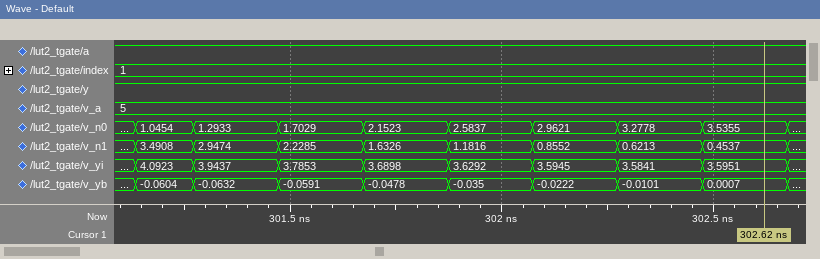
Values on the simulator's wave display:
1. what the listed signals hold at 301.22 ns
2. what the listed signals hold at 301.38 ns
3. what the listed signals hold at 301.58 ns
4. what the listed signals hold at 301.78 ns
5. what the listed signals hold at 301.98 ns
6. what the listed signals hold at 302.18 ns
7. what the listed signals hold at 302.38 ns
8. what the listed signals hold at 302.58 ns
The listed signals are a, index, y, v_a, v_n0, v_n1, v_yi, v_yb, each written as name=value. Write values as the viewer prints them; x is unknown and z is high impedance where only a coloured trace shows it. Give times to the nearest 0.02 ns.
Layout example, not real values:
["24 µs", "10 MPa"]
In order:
["a=1, index=1, y=1, v_a=5, v_n0=1.0454, v_n1=3.4908, v_yi=4.0923, v_yb=-0.0604", "a=1, index=1, y=1, v_a=5, v_n0=1.2933, v_n1=2.9474, v_yi=3.9437, v_yb=-0.0632", "a=1, index=1, y=1, v_a=5, v_n0=1.7029, v_n1=2.2285, v_yi=3.7853, v_yb=-0.0591", "a=1, index=1, y=1, v_a=5, v_n0=2.1523, v_n1=1.6326, v_yi=3.6898, v_yb=-0.0478", "a=1, index=1, y=1, v_a=5, v_n0=2.5837, v_n1=1.1816, v_yi=3.6292, v_yb=-0.035", "a=1, index=1, y=1, v_a=5, v_n0=2.9621, v_n1=0.8552, v_yi=3.5945, v_yb=-0.0222", "a=1, index=1, y=1, v_a=5, v_n0=3.2778, v_n1=0.6213, v_yi=3.5841, v_yb=-0.0101", "a=1, index=1, y=1, v_a=5, v_n0=3.5355, v_n1=0.4537, v_yi=3.5951, v_yb=0.0007"]
